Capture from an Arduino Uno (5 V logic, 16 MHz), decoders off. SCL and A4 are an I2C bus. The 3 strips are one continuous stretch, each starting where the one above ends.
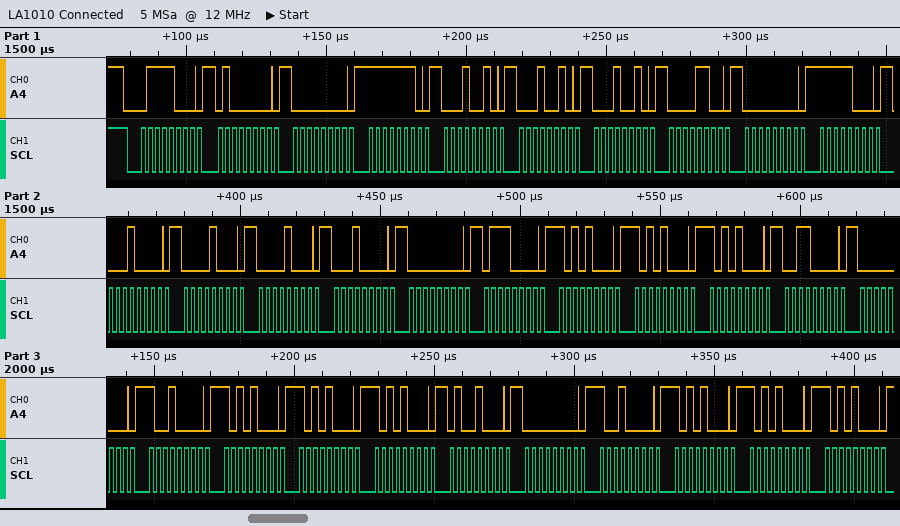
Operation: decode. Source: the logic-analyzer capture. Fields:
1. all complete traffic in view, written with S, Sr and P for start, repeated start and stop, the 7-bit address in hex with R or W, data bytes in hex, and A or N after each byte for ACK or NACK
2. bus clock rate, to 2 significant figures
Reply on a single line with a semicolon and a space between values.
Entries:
S 3CW A 40 A 00 A FE A 12 A 12 A 12 A 0C A 00 A F8 A 10 A 08 A 08 A 10 A 00 A 70 A A8 A A8 A A8 A 30 A 00 A 90 A A8 A A8 A A8 A 48 A 00 A 90 A A8 A A8 A A8 A; 400 kHz
